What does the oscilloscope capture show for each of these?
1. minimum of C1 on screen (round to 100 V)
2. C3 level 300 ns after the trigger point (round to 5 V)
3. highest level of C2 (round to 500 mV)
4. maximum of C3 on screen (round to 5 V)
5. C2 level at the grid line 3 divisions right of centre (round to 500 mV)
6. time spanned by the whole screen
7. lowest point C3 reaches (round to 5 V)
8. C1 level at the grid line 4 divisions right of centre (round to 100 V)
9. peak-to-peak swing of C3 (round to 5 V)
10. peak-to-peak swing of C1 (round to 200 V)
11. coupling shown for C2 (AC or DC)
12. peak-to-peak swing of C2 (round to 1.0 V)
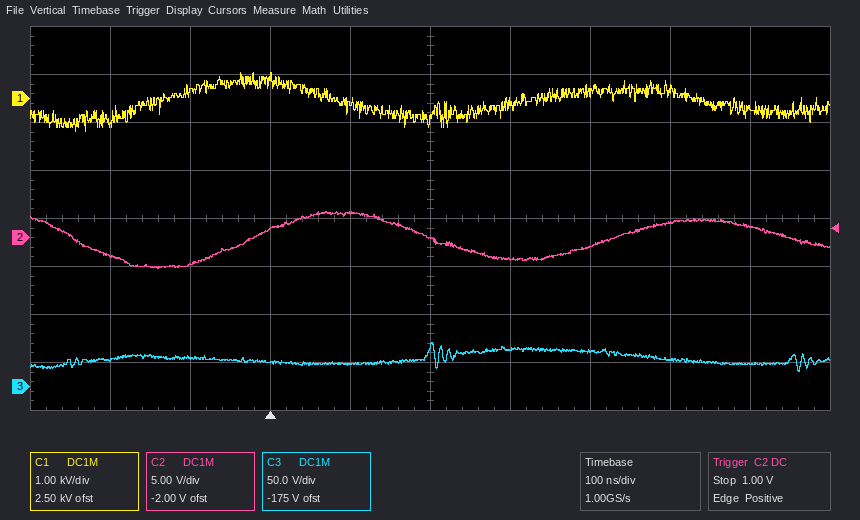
-700 V
40 V
2.5 V
45 V
1.5 V
1 µs
15 V
-200 V
30 V
1.2 kV
DC
6.0 V
